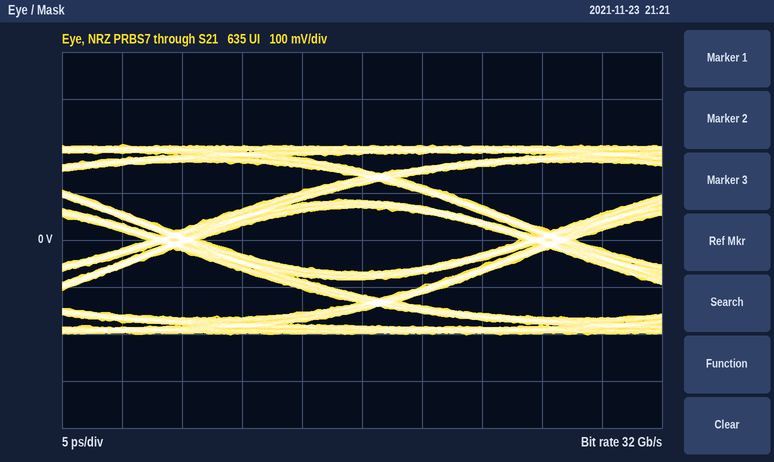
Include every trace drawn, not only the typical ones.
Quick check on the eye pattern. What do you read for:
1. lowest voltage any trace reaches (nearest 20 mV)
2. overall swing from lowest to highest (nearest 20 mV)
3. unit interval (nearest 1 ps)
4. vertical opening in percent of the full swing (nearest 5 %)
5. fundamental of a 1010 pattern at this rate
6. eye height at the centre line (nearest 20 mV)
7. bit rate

-200 mV
400 mV
31 ps
35 %
16 GHz
140 mV
32 Gb/s
